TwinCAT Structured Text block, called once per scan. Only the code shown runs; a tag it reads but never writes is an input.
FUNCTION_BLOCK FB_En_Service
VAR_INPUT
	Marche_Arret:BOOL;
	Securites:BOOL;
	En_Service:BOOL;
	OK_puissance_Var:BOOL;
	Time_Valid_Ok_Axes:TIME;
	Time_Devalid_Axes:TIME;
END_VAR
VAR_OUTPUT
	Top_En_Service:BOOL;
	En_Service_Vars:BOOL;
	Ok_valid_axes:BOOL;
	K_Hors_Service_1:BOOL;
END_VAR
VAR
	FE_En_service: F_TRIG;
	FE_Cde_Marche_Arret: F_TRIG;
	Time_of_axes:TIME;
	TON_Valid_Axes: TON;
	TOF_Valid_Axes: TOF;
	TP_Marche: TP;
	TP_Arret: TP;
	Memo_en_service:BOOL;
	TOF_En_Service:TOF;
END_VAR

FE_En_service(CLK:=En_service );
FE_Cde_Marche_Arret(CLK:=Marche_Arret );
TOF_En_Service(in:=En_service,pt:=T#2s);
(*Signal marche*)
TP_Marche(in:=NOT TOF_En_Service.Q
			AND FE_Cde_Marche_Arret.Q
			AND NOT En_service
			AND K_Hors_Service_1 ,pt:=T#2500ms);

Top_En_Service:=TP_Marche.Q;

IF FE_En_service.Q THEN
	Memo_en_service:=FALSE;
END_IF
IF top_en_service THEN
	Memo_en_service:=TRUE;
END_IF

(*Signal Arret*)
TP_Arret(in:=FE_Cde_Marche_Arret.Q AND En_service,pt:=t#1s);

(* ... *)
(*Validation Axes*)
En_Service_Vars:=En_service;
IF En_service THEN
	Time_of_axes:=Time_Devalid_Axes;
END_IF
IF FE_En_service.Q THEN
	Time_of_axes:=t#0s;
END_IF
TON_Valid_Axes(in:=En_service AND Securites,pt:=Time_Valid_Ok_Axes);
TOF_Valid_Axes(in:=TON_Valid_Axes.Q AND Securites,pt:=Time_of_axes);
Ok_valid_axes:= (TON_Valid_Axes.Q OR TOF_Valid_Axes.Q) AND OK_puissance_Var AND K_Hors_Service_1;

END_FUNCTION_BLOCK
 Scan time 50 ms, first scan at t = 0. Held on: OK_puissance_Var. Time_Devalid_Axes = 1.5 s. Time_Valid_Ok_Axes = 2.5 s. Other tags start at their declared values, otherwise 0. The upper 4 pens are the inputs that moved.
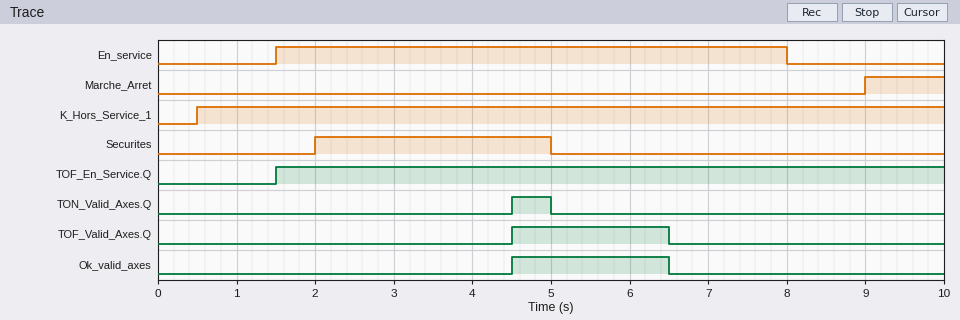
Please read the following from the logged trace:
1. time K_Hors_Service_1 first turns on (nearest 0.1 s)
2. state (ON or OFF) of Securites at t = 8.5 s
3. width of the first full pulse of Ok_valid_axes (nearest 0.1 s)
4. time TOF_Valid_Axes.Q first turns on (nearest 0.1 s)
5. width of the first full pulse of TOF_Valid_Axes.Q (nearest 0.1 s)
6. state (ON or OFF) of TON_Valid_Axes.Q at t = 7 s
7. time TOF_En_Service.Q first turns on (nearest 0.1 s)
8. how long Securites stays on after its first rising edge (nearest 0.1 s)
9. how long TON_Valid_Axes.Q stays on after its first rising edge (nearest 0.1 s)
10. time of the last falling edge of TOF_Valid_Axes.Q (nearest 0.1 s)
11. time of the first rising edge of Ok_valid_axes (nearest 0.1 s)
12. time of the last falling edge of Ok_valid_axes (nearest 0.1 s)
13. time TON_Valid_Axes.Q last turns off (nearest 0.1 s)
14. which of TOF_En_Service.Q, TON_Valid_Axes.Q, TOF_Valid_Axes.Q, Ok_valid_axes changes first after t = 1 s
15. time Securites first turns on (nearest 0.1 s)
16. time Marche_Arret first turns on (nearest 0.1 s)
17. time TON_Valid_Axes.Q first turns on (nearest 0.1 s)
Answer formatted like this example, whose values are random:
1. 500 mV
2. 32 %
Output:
1. 0.5 s
2. OFF
3. 2.0 s
4. 4.5 s
5. 2.0 s
6. OFF
7. 1.5 s
8. 3.0 s
9. 0.5 s
10. 6.5 s
11. 4.5 s
12. 6.5 s
13. 5.0 s
14. TOF_En_Service.Q
15. 2.0 s
16. 9.0 s
17. 4.5 s
